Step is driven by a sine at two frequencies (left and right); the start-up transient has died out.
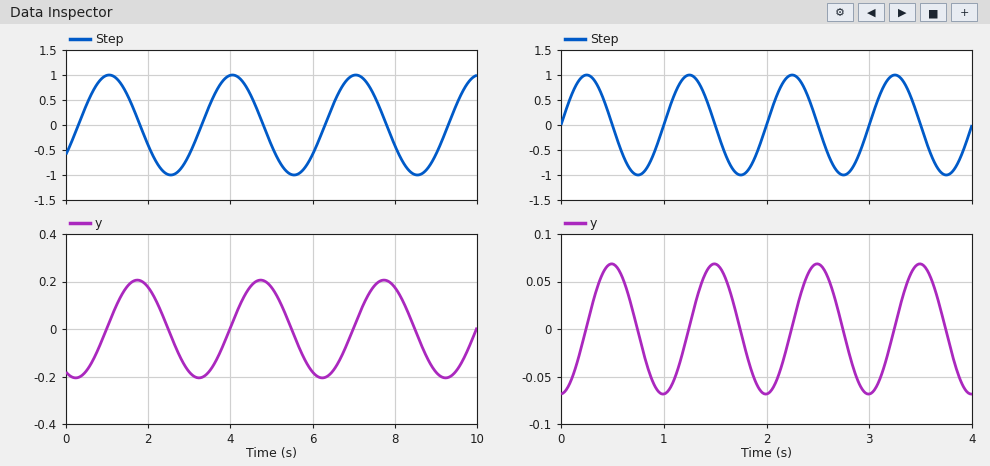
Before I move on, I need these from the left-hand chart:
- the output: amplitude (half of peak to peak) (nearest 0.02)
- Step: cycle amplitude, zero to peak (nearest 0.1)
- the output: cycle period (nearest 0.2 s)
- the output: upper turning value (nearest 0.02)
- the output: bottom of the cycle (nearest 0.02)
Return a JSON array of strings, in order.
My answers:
["0.20", "1.0", "3.0 s", "0.20", "-0.20"]
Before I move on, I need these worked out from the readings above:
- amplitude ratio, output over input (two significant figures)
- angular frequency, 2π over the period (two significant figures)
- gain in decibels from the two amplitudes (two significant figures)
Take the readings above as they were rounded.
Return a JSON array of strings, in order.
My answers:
["0.20", "2.1 rad/s", "-14 dB"]
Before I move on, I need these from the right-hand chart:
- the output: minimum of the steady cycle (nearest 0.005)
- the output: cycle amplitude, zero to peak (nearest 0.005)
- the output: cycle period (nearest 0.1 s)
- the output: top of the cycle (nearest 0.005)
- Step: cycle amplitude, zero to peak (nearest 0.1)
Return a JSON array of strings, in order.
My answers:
["-0.070", "0.070", "1.0 s", "0.070", "1.0"]
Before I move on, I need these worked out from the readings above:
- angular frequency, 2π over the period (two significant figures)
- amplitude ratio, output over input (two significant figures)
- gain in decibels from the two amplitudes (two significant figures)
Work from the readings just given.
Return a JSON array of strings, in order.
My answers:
["6.3 rad/s", "0.070", "-23 dB"]
